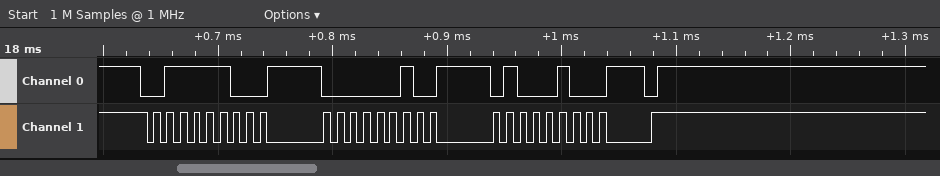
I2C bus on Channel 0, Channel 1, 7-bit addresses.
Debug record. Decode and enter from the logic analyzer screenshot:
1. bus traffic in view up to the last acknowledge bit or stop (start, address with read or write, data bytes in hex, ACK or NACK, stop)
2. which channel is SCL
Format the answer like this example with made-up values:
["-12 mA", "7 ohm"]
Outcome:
["start, address 3E write ACK, 02 ACK, 44 ACK, stop", "Channel 1"]
